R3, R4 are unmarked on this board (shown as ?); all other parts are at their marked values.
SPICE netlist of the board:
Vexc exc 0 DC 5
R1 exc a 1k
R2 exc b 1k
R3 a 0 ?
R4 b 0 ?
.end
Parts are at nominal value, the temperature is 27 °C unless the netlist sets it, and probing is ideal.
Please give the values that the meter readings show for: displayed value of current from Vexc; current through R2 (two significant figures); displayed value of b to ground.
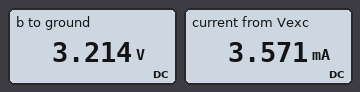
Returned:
3.571 mA
1.8 mA
3.214 V
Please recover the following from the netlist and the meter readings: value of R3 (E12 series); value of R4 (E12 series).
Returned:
1.8 kΩ
1.8 kΩ
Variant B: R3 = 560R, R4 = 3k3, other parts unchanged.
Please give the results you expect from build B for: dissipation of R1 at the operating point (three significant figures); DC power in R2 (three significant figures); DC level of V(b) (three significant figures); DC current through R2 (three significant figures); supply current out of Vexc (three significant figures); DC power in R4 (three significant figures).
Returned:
10.3 mW
1.35 mW
3.84 V
1.16 mA
4.37 mA
4.46 mW
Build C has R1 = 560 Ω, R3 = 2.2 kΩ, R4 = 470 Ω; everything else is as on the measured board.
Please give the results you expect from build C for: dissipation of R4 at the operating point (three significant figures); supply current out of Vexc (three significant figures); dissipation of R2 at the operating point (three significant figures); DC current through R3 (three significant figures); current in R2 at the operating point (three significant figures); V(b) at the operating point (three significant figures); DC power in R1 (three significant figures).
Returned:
5.44 mW
5.21 mA
11.6 mW
1.81 mA
3.40 mA
1.60 V
1.84 mW
